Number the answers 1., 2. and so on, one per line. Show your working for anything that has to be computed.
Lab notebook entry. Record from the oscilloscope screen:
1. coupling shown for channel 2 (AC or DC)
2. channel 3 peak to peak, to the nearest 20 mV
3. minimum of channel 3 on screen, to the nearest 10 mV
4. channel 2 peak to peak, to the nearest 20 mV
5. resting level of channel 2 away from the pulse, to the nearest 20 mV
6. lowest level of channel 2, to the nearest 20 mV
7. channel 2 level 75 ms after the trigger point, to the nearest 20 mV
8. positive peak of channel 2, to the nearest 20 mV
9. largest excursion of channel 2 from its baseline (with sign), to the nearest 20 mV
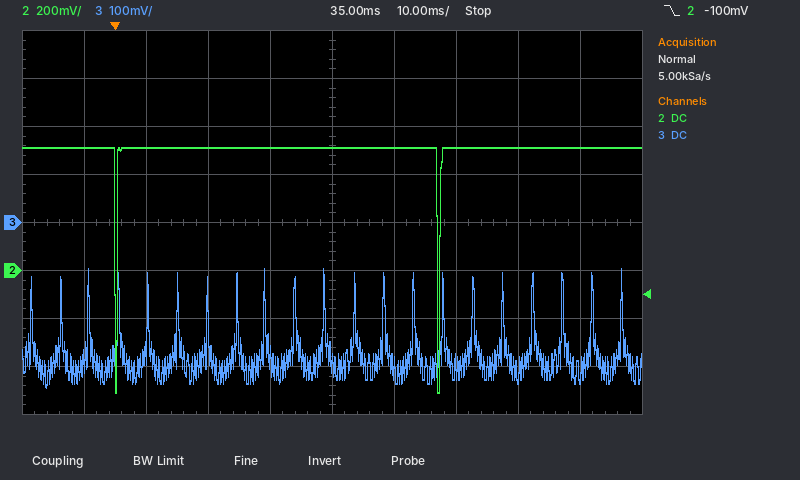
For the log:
1. DC
2. 240 mV
3. -340 mV
4. 520 mV − (-500 mV) = 1.02 V
5. 520 mV
6. -500 mV
7. 520 mV
8. 520 mV
9. -500 mV − (520 mV) = -1.02 V
